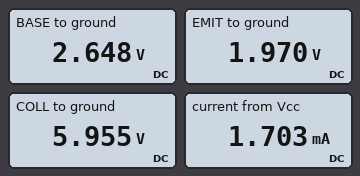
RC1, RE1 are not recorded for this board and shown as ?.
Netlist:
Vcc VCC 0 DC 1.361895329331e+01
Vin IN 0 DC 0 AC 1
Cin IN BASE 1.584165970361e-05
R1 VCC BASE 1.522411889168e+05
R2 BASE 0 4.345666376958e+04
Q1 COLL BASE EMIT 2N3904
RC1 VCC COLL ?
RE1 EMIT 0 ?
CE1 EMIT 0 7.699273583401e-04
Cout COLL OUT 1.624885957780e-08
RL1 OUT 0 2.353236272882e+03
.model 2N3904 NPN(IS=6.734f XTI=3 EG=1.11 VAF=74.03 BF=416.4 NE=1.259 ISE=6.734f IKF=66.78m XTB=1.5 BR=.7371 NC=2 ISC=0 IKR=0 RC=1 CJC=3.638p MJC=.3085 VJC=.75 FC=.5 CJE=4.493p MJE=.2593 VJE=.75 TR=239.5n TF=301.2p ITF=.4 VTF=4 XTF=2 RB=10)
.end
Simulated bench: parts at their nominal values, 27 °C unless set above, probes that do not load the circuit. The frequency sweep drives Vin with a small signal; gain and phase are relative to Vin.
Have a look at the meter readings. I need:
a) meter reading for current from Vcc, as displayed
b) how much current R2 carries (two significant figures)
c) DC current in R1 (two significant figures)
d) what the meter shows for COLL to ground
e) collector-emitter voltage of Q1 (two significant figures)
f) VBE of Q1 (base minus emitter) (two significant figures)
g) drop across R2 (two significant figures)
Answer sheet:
1.703 mA
61 µA
72 µA
5.955 V
4.0 V
680 mV
2.6 V
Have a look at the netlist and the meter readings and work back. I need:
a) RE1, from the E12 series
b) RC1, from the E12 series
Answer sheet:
1.2 kΩ
4.7 kΩ
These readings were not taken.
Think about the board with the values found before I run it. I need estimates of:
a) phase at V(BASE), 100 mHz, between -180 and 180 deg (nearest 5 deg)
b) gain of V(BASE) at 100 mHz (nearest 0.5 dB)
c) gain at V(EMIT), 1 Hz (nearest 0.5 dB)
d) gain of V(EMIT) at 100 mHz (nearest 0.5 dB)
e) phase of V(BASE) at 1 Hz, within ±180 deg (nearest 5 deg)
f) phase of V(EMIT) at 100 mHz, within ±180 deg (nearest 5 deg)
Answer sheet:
70 deg
-11.5 dB
-3.0 dB
-11.5 dB
15 deg
70 deg
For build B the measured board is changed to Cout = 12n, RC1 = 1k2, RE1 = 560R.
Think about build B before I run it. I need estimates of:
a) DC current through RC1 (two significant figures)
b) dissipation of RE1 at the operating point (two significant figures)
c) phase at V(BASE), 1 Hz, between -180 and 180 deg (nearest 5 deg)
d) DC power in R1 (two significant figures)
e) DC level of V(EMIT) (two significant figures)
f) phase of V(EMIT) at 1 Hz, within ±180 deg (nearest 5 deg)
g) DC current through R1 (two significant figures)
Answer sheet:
3.0 mA
5.2 mW
20 deg
830 µW
1.7 V
15 deg
74 µA
